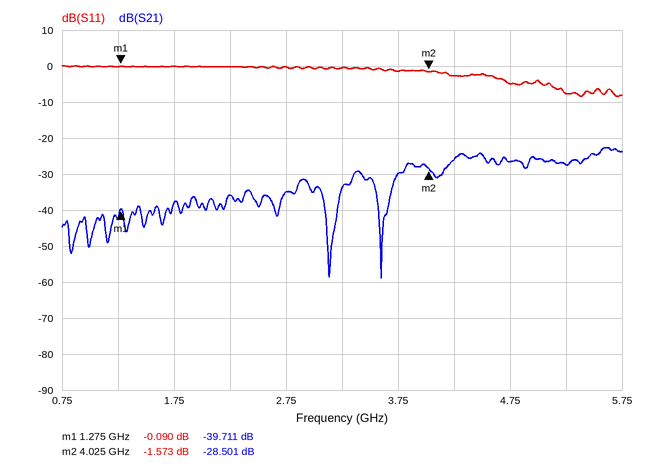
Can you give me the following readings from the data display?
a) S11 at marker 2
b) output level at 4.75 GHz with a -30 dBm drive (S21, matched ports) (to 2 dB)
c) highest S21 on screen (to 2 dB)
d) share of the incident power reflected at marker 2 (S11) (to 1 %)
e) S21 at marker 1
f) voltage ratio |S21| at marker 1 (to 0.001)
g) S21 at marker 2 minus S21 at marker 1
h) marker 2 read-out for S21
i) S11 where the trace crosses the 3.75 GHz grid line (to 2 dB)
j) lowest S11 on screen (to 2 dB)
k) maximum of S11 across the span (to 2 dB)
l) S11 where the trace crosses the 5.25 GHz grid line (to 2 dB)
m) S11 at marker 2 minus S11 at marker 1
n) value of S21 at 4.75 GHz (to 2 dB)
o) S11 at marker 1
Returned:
-1.573 dB
-56 dBm
-22 dB
70 %
-39.711 dB
0.010
11.210 dB
-28.501 dB
-2 dB
-8 dB
0 dB
-8 dB
-1.483 dB
-26 dB
-0.090 dB
